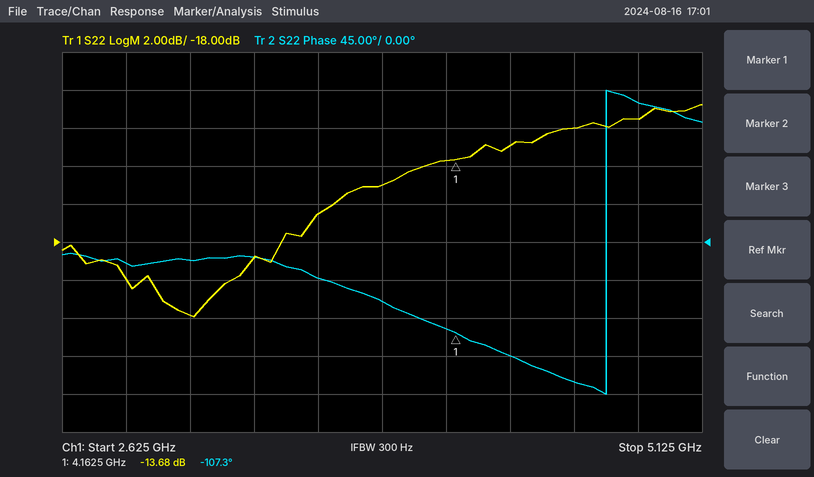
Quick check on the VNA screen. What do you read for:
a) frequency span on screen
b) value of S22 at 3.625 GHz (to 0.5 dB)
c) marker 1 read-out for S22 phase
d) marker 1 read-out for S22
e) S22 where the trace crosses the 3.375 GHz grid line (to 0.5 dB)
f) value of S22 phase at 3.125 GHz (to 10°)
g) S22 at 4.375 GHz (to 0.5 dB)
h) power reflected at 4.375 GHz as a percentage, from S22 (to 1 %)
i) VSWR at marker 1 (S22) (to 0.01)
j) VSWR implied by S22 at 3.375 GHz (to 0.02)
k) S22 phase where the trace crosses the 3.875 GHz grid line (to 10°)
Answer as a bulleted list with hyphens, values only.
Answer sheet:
- 2.5 GHz
- -16.5 dB
- -107.3°
- -13.68 dB
- -19.0 dB
- -20°
- -13.0 dB
- 5 %
- 1.52
- 1.26
- -70°
